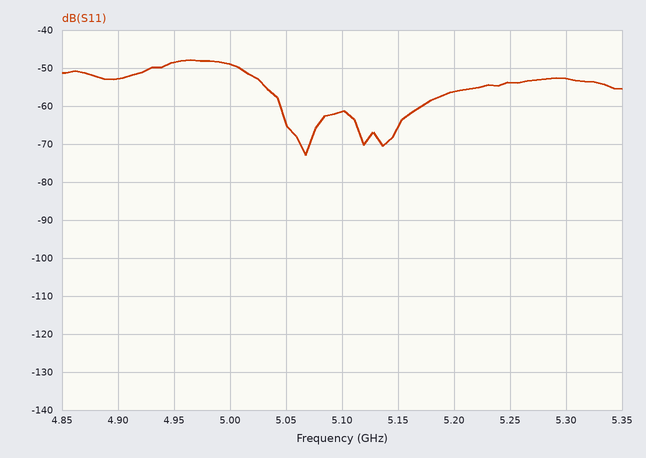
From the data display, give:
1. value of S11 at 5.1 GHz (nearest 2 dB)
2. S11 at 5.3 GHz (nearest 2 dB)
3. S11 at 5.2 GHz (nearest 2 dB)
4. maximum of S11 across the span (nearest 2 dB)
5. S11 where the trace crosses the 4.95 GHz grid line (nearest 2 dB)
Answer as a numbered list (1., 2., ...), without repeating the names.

1. -62 dB
2. -52 dB
3. -56 dB
4. -48 dB
5. -48 dB
